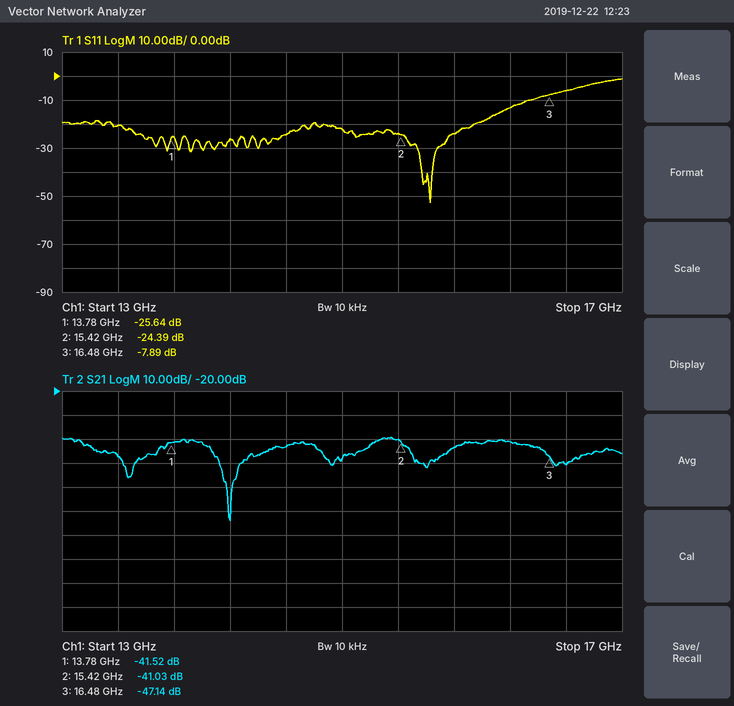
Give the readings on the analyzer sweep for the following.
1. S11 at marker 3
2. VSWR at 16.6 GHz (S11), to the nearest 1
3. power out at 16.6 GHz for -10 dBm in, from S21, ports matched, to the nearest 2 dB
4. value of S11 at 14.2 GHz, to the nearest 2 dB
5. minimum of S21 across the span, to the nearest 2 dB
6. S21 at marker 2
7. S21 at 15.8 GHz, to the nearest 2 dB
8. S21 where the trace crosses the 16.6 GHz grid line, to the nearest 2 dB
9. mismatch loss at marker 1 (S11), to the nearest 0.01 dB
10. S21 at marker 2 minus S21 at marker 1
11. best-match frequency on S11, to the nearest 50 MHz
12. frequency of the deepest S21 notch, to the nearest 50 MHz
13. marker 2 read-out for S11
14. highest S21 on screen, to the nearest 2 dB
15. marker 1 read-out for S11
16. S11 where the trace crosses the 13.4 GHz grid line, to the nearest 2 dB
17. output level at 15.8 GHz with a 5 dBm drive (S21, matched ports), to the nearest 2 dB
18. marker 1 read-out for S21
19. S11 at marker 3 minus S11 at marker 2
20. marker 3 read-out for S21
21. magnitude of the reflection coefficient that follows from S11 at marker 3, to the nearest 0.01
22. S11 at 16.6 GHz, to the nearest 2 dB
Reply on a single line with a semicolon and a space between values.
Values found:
-7.89 dB; 3; -60 dBm; -26 dB; -74 dB; -41.03 dB; -44 dB; -50 dB; 0.01 dB; 0.49 dB; 15.65 GHz; 14.20 GHz; -24.39 dB; -40 dB; -25.64 dB; -20 dB; -38 dBm; -41.52 dB; 16.50 dB; -47.14 dB; 0.40; -6 dB
